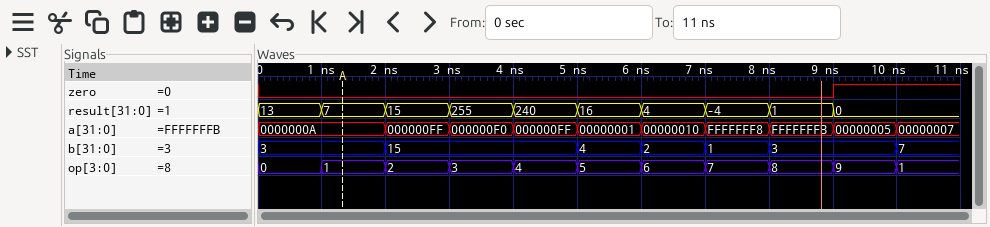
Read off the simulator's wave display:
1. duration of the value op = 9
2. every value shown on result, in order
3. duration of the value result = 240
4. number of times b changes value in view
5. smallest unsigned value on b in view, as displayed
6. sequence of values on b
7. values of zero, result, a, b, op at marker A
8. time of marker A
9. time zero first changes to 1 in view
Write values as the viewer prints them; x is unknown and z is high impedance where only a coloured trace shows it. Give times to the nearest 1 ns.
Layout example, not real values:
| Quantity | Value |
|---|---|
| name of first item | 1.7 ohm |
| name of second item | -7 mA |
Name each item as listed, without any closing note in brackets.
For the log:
| Quantity | Value |
|---|---|
| duration of the value op = 9 | 1 ns |
| every value shown on result, in order | 13, 7, 15, 255, 240, 16, 4, -4, 1, 0 |
| duration of the value result = 240 | 1 ns |
| number of times b changes value in view | 6 |
| smallest unsigned value on b in view, as displayed | 1 |
| sequence of values on b | 3, 15, 4, 2, 1, 3, 7 |
| values of zero, result, a, b, op at marker A | zero=0, result=7, a=0000000A, b=3, op=1 |
| time of marker A | 1 ns |
| time zero first changes to 1 in view | 9 ns |
